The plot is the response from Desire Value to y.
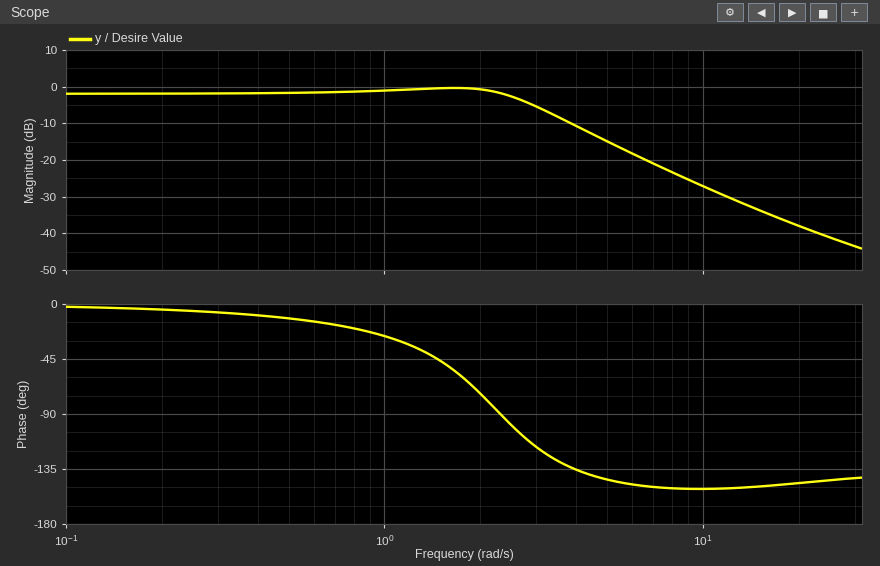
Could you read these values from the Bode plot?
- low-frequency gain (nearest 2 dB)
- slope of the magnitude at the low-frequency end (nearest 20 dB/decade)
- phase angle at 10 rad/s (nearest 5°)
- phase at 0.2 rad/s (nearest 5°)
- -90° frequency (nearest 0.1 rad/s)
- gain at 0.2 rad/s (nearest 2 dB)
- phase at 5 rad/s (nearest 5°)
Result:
-2 dB
0 dB/decade
-150°
-5°
2.3 rad/s
-2 dB
-145°
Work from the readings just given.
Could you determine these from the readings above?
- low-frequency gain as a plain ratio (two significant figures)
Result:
0.79
